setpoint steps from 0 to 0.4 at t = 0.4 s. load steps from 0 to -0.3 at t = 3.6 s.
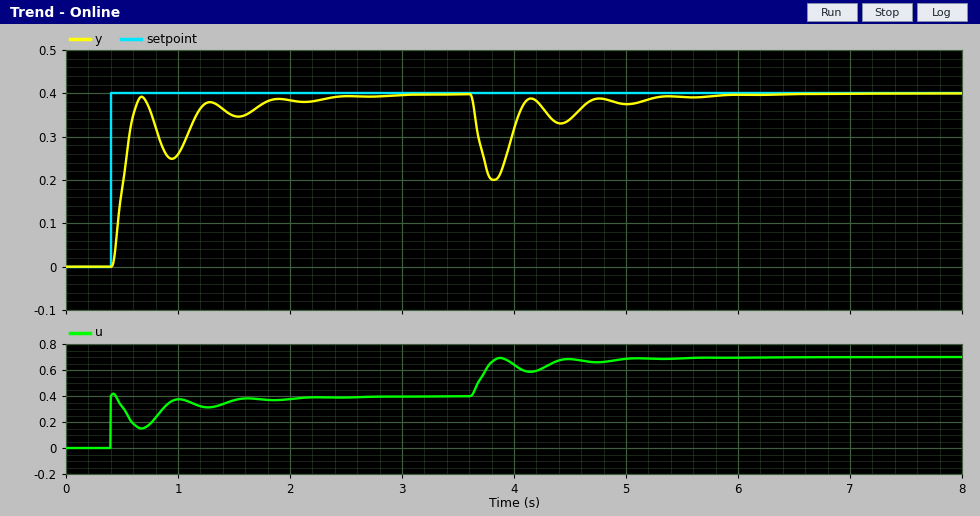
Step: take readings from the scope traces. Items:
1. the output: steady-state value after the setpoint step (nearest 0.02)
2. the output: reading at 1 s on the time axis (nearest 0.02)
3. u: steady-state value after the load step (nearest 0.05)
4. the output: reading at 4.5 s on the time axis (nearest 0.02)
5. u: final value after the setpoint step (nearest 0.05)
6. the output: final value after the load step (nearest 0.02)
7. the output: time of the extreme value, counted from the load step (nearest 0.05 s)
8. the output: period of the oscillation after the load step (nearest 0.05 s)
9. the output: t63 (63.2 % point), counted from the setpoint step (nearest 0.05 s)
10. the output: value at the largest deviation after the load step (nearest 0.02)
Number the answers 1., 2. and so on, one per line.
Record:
1. 0.40
2. 0.26
3. 0.70
4. 0.34
5. 0.40
6. 0.40
7. 0.20 s
8. 0.60 s
9. 0.15 s
10. 0.20
